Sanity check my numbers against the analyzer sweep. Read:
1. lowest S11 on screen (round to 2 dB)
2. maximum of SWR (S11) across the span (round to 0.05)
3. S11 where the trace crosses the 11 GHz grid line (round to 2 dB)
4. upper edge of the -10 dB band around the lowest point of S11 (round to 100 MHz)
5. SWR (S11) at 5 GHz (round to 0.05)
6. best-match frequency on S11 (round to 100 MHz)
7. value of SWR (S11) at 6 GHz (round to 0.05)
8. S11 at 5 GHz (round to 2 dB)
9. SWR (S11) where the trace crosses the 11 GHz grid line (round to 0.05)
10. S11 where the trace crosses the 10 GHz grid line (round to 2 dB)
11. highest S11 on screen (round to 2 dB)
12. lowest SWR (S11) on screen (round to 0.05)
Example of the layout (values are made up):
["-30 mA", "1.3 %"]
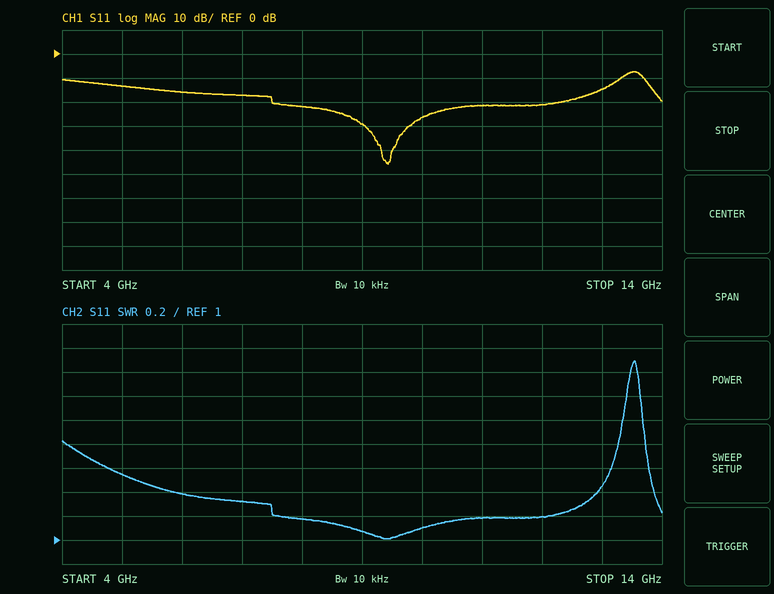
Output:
["-46 dB", "2.50", "-22 dB", "13.3 GHz", "1.55", "9.4 GHz", "1.40", "-14 dB", "1.20", "-26 dB", "-8 dB", "1.00"]
